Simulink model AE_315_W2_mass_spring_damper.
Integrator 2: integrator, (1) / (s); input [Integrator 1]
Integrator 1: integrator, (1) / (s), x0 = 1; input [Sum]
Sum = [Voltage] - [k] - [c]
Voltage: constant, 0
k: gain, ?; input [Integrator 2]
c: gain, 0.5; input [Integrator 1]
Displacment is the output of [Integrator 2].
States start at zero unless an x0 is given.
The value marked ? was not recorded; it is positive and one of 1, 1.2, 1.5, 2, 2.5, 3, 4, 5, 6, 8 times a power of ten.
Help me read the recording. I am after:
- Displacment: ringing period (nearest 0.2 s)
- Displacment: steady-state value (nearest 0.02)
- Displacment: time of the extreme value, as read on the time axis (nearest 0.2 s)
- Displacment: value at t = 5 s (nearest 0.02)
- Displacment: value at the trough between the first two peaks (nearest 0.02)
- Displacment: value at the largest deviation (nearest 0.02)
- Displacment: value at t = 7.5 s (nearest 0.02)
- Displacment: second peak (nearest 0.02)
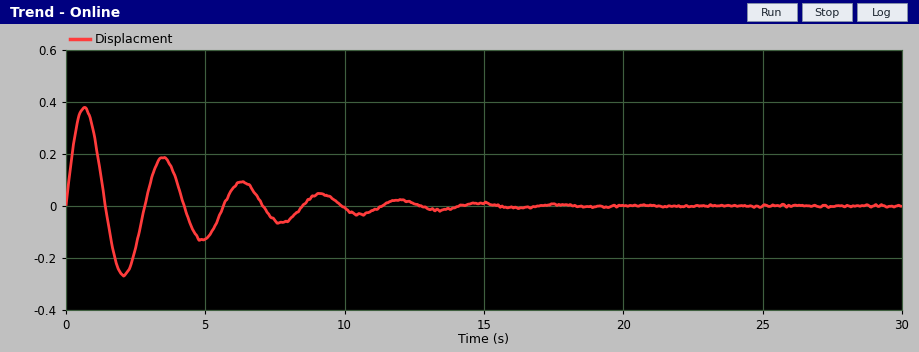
2.8 s
0.00
0.6 s
-0.12
-0.26
0.38
-0.06
0.18
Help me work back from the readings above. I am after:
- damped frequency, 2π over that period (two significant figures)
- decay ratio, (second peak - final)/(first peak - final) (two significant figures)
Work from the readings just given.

2.2 rad/s
0.47
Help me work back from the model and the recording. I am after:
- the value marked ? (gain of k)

5
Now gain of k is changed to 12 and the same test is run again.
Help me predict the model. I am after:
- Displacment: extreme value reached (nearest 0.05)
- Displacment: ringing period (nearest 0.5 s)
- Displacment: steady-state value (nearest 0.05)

0.25
2.0 s
0.00
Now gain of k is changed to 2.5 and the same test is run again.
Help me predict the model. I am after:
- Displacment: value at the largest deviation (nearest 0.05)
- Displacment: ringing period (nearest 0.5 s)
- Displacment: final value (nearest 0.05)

0.50
4.0 s
0.00
